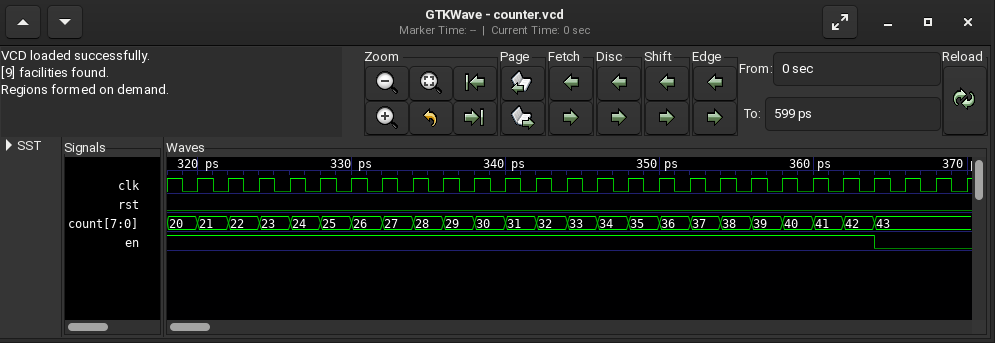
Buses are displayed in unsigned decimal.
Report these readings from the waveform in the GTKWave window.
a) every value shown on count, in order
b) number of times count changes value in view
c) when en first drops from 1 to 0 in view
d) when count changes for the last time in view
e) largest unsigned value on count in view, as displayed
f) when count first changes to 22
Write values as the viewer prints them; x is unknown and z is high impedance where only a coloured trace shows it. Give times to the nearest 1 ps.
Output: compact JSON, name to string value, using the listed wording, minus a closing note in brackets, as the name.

{"every value shown on count, in order": "20, 21, 22, 23, 24, 25, 26, 27, 28, 29, 30, 31, 32, 33, 34, 35, 36, 37, 38, 39, 40, 41, 42, 43", "number of times count changes value in view": "23", "when en first drops from 1 to 0 in view": "364 ps", "when count changes for the last time in view": "364 ps", "largest unsigned value on count in view, as displayed": "43", "when count first changes to 22": "322 ps"}
